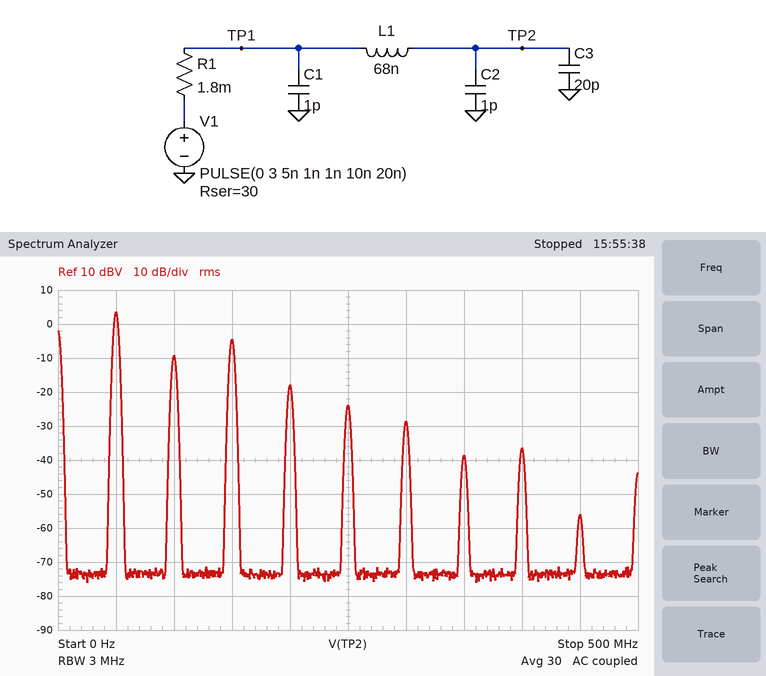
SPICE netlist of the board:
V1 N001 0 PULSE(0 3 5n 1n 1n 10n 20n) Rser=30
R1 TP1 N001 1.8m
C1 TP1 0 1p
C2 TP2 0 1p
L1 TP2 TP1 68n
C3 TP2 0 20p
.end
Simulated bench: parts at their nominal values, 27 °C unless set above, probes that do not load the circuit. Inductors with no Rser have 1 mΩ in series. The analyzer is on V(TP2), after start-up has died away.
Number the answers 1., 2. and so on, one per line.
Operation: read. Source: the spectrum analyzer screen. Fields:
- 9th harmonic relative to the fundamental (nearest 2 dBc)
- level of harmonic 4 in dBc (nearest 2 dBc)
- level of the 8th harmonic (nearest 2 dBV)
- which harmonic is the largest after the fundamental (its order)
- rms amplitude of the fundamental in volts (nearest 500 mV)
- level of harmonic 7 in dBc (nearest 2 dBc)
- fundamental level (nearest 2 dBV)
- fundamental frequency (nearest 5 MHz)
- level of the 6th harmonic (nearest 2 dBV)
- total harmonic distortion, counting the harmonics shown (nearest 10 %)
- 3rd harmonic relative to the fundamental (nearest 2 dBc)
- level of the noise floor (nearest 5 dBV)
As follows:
1. -60 dBc
2. -22 dBc
3. -36 dBV
4. 3
5. 1.5 V
6. -42 dBc
7. 4 dBV
8. 50 MHz
9. -28 dBV
10. 50 %
11. -8 dBc
12. -75 dBV
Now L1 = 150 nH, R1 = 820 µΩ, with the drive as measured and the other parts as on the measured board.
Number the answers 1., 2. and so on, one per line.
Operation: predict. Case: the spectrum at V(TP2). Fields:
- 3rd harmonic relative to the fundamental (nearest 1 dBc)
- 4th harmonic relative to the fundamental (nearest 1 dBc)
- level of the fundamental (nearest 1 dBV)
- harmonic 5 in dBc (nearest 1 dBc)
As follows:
1. -19 dBc
2. -32 dBc
3. 5 dBV
4. -37 dBc
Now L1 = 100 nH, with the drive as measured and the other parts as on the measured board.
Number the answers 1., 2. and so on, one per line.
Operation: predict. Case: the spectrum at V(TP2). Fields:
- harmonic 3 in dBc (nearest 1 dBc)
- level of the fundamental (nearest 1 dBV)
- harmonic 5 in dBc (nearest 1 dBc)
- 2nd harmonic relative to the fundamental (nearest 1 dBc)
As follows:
1. -13 dBc
2. 4 dBV
3. -32 dBc
4. -11 dBc
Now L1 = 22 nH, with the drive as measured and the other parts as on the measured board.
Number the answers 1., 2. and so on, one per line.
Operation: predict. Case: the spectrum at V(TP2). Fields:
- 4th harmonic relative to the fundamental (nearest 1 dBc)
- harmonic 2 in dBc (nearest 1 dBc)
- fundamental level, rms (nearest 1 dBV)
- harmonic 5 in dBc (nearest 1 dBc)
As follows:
1. -16 dBc
2. -16 dBc
3. 3 dBV
4. -18 dBc
